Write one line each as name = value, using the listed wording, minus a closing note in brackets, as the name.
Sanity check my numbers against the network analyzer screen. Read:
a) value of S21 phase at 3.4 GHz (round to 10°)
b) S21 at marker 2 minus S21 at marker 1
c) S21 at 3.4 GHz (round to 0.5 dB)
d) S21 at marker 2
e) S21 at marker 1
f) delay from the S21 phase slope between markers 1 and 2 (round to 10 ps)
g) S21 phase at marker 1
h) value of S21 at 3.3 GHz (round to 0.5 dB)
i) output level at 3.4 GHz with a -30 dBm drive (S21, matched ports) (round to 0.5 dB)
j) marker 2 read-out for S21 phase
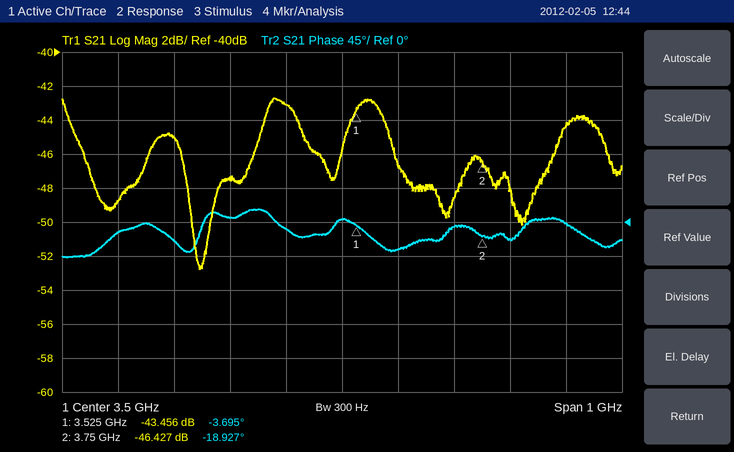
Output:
value of S21 phase at 3.4 GHz = -10°
S21 at marker 2 minus S21 at marker 1 = -2.971 dB
S21 at 3.4 GHz = -43.0 dB
S21 at marker 2 = -46.427 dB
S21 at marker 1 = -43.456 dB
delay from the S21 phase slope between markers 1 and 2 = 190 ps
S21 phase at marker 1 = -3.695°
value of S21 at 3.3 GHz = -47.5 dB
output level at 3.4 GHz with a -30 dBm drive (S21, matched ports) = -73.0 dBm
marker 2 read-out for S21 phase = -18.927°
